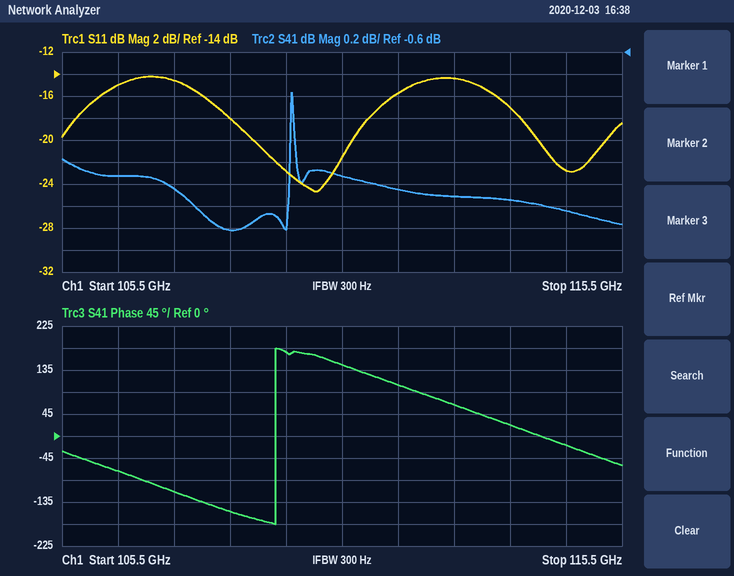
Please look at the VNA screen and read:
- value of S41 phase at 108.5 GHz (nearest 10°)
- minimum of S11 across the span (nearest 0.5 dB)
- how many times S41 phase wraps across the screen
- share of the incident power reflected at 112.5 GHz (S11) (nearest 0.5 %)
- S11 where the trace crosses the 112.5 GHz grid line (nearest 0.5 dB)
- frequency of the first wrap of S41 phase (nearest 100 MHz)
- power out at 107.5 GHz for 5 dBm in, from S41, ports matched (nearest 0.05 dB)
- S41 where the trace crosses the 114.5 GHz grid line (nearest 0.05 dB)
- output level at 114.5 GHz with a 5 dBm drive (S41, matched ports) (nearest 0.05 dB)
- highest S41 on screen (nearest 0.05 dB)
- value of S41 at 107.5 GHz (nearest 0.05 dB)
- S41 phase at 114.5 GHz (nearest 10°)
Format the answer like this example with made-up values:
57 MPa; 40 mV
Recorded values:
-150°; -24.5 dB; 1; 3.5 %; -14.5 dB; 109.3 GHz; 3.15 dBm; -2.05 dB; 2.95 dBm; -0.95 dB; -1.85 dB; -20°
